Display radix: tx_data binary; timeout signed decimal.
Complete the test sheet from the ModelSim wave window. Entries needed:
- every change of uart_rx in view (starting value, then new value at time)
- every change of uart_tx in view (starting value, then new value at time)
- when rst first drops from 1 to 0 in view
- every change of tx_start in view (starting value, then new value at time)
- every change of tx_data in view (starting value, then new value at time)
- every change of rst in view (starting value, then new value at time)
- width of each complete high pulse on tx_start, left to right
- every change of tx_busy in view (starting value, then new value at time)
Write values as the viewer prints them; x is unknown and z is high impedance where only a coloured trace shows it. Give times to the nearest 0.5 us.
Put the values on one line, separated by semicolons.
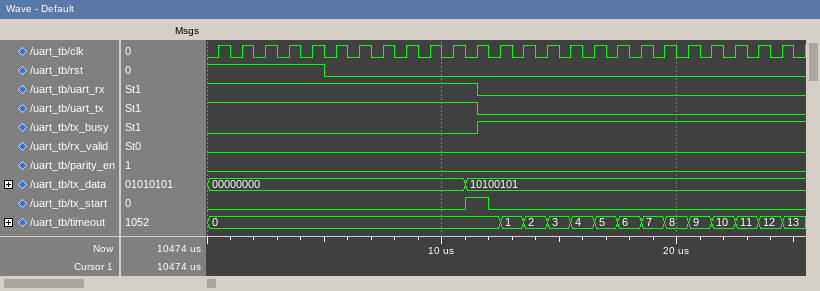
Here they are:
1, 0 at 11.5 us; 1, 0 at 11.5 us; 5 us; 0, 1 at 11 us, 0 at 12 us; 00000000, 10100101 at 11 us; 1, 0 at 5 us; 1 us; 0, 1 at 11.5 us
